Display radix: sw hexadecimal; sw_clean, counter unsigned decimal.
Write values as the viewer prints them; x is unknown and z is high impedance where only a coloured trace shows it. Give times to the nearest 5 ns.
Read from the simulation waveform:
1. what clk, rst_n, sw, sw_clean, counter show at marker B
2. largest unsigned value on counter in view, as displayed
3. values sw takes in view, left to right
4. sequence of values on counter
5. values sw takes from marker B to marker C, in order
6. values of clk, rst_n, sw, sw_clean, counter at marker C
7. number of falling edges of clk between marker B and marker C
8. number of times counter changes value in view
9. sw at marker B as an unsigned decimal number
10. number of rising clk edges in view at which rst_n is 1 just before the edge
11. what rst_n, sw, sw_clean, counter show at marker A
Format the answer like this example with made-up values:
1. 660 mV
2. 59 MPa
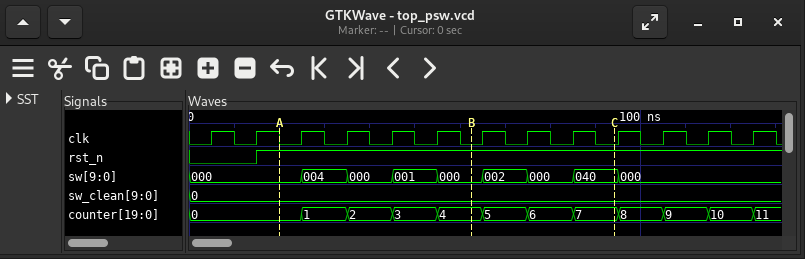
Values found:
1. clk=0, rst_n=1, sw=000, sw_clean=0, counter=4
2. 11
3. 000, 004, 000, 001, 000, 002, 000, 040, 000
4. 0, 1, 2, 3, 4, 5, 6, 7, 8, 9, 10, 11
5. 000, 002, 000, 040
6. clk=0, rst_n=1, sw=040, sw_clean=0, counter=7
7. 3
8. 11
9. 0
10. 11
11. rst_n=1, sw=000, sw_clean=0, counter=0
